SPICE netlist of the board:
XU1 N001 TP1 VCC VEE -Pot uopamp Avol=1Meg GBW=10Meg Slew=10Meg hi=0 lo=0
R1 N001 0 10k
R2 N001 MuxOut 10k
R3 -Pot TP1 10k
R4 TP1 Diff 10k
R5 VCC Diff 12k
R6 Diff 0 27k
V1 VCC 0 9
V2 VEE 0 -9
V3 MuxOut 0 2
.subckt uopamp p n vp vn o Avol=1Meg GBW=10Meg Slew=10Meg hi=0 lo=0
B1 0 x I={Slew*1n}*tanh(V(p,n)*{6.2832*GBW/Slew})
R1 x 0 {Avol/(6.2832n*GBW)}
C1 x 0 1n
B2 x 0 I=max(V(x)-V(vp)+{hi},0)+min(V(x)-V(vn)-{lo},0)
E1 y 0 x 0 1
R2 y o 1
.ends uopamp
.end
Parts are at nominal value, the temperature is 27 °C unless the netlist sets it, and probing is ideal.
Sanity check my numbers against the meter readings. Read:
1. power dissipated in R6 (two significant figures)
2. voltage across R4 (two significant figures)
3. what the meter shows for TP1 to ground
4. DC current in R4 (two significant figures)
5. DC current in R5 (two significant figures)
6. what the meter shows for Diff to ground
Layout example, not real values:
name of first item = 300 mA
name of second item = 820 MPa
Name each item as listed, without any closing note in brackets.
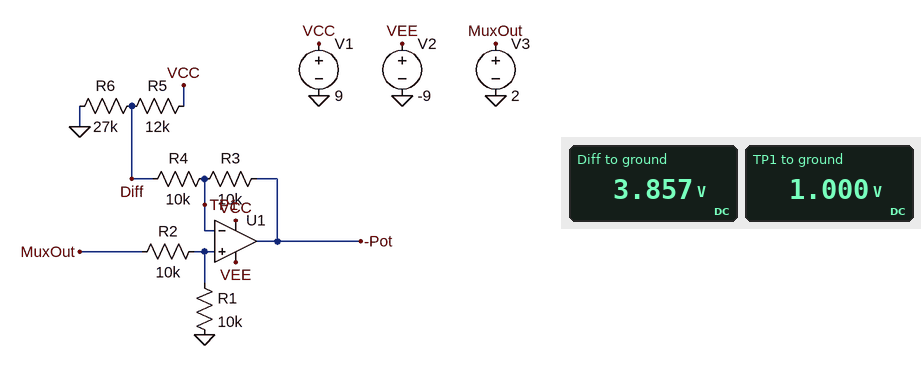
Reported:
power dissipated in R6 = 550 µW
voltage across R4 = 2.9 V
what the meter shows for TP1 to ground = 1.000 V
DC current in R4 = 290 µA
DC current in R5 = 430 µA
what the meter shows for Diff to ground = 3.857 V
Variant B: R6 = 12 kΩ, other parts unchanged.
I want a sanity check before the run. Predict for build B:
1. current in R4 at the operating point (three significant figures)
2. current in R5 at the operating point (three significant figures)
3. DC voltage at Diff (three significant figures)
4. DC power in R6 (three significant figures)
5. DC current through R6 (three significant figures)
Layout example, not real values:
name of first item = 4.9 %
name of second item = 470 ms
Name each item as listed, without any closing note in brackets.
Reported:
current in R4 at the operating point = 219 µA
current in R5 at the operating point = 484 µA
DC voltage at Diff = 3.19 V
DC power in R6 = 847 µW
DC current through R6 = 266 µA
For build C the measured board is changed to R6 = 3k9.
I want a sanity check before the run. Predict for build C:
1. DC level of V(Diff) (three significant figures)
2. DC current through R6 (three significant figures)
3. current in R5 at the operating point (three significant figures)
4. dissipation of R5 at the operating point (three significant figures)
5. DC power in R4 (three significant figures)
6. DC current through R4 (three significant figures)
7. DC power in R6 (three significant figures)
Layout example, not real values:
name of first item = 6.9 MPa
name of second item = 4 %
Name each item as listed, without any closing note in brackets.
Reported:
DC level of V(Diff) = 1.93 V
DC current through R6 = 496 µA
current in R5 at the operating point = 589 µA
dissipation of R5 at the operating point = 4.16 mW
DC power in R4 = 87.0 µW
DC current through R4 = 93.3 µA
DC power in R6 = 958 µW
